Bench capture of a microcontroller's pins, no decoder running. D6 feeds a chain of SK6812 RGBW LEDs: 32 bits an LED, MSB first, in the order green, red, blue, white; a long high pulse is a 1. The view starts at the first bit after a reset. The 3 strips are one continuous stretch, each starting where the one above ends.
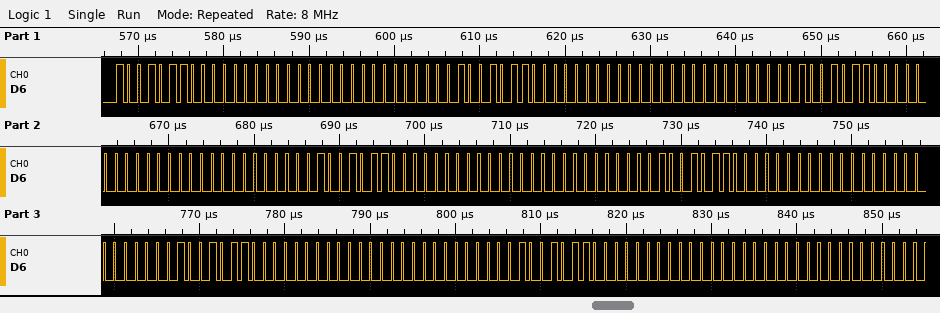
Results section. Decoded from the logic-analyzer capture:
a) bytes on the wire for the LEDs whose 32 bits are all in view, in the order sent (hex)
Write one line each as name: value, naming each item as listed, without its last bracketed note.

bytes on the wire for the LEDs whose 32 bits are all in view, in the order sent: 96 00 00 00 96 00 00 00 96 00 00 00 96 00 00 00 96 00 00 00 96 00 00 00 96 00 00 00
